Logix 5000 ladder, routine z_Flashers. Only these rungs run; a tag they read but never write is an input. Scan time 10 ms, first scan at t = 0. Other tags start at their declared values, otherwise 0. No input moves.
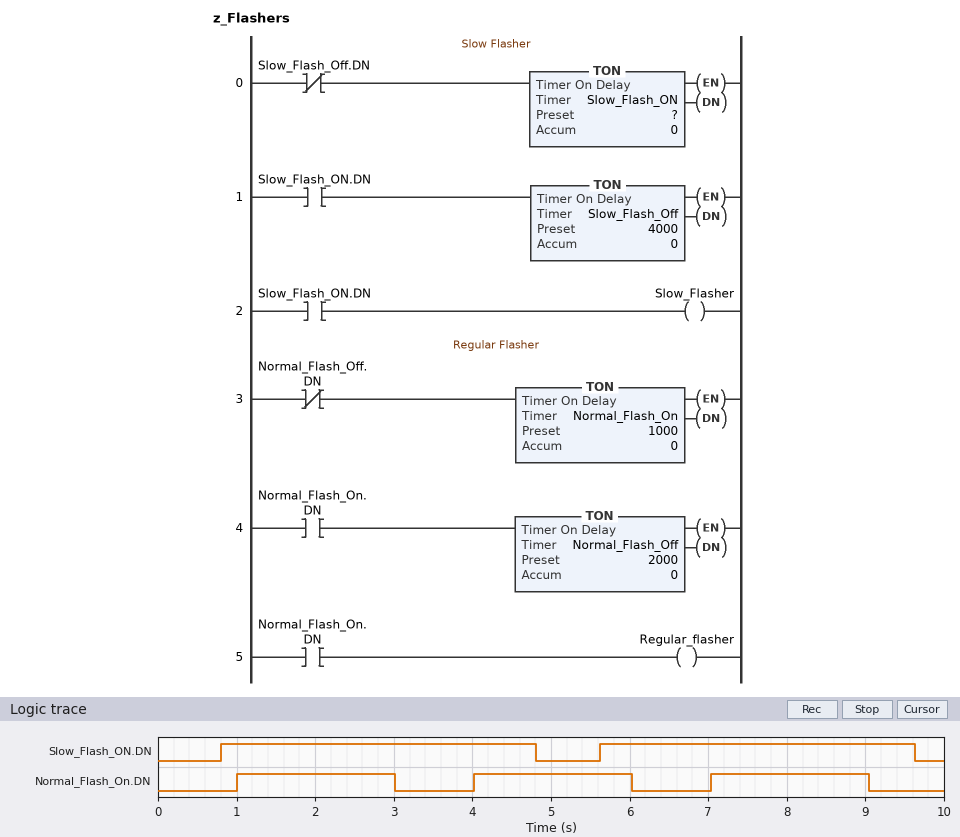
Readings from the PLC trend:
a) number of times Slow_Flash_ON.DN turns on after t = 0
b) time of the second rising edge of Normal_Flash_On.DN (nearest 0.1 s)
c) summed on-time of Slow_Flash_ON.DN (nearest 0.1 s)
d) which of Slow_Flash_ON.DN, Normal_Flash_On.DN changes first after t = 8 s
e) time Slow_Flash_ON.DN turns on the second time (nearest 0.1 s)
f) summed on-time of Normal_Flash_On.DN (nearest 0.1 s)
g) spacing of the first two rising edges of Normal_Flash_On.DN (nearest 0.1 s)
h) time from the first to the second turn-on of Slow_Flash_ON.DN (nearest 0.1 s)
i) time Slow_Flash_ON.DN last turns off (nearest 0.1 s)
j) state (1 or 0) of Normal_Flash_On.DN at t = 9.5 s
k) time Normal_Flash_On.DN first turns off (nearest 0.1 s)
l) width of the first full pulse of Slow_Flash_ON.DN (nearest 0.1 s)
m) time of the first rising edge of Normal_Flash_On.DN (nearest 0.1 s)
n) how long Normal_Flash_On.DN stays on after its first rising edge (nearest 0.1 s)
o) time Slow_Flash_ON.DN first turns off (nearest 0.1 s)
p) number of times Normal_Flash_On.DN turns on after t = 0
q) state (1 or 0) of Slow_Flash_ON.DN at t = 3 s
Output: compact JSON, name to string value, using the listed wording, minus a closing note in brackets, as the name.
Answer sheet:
{"number of times Slow_Flash_ON.DN turns on after t = 0": "2", "time of the second rising edge of Normal_Flash_On.DN": "4.0 s", "summed on-time of Slow_Flash_ON.DN": "8.0 s", "which of Slow_Flash_ON.DN, Normal_Flash_On.DN changes first after t = 8 s": "Normal_Flash_On.DN", "time Slow_Flash_ON.DN turns on the second time": "5.6 s", "summed on-time of Normal_Flash_On.DN": "6.0 s", "spacing of the first two rising edges of Normal_Flash_On.DN": "3.0 s", "time from the first to the second turn-on of Slow_Flash_ON.DN": "4.8 s", "time Slow_Flash_ON.DN last turns off": "9.6 s", "state (1 or 0) of Normal_Flash_On.DN at t = 9.5 s": "0", "time Normal_Flash_On.DN first turns off": "3.0 s", "width of the first full pulse of Slow_Flash_ON.DN": "4.0 s", "time of the first rising edge of Normal_Flash_On.DN": "1.0 s", "how long Normal_Flash_On.DN stays on after its first rising edge": "2.0 s", "time Slow_Flash_ON.DN first turns off": "4.8 s", "number of times Normal_Flash_On.DN turns on after t = 0": "3", "state (1 or 0) of Slow_Flash_ON.DN at t = 3 s": "1"}
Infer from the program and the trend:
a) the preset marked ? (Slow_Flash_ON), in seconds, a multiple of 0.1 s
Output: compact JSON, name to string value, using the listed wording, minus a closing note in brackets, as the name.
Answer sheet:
{"the preset marked ? (Slow_Flash_ON), in seconds, a multiple of 0.1 s": "0.8 s"}
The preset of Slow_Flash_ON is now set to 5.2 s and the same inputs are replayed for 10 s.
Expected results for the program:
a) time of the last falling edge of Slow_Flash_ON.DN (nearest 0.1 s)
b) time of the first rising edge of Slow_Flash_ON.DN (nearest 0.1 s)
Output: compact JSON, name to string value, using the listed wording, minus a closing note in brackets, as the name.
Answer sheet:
{"time of the last falling edge of Slow_Flash_ON.DN": "9.2 s", "time of the first rising edge of Slow_Flash_ON.DN": "5.2 s"}
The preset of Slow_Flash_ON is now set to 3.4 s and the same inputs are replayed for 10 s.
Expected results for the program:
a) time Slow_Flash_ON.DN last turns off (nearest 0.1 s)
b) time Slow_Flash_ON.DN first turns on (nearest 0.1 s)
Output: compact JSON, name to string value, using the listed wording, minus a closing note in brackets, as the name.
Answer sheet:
{"time Slow_Flash_ON.DN last turns off": "7.4 s", "time Slow_Flash_ON.DN first turns on": "3.4 s"}
